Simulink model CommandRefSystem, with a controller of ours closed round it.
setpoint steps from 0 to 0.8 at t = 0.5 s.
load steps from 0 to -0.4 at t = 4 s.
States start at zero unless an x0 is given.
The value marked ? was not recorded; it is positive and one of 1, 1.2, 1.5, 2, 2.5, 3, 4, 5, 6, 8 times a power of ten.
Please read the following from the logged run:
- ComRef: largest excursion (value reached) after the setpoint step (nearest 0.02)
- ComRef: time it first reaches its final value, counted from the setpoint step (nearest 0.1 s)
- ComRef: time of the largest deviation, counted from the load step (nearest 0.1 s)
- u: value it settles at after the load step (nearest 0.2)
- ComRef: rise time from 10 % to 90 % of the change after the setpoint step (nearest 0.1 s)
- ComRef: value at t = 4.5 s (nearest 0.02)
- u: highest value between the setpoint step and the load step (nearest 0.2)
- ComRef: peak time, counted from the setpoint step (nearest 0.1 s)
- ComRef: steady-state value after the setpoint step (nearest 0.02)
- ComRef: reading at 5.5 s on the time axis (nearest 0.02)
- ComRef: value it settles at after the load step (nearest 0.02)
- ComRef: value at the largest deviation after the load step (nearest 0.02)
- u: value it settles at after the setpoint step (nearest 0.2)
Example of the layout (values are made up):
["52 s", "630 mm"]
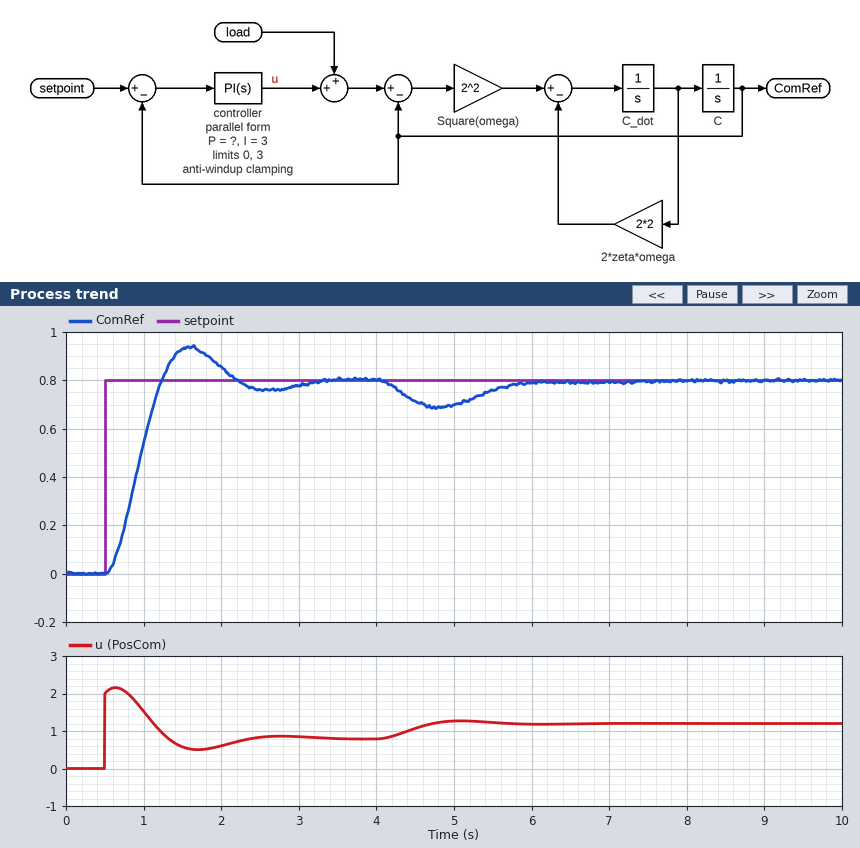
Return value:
["0.94", "0.7 s", "0.8 s", "1.2", "0.5 s", "0.72", "2.2", "1.1 s", "0.80", "0.76", "0.80", "0.68", "0.8"]
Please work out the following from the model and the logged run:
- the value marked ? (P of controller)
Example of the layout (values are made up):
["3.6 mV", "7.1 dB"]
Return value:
["2.5"]
